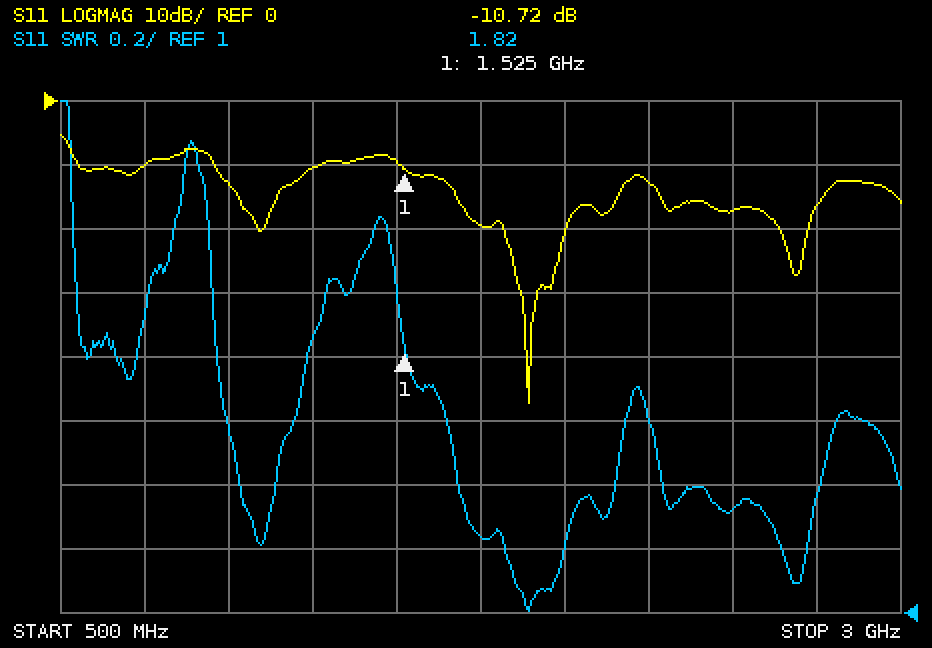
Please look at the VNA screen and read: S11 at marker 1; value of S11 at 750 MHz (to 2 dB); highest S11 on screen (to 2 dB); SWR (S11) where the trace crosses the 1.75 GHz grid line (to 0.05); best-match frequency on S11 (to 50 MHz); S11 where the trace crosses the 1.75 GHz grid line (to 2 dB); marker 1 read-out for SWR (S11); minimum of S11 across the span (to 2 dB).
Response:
-10.72 dB
-10 dB
-6 dB
1.25
1.90 GHz
-20 dB
1.82
-48 dB
